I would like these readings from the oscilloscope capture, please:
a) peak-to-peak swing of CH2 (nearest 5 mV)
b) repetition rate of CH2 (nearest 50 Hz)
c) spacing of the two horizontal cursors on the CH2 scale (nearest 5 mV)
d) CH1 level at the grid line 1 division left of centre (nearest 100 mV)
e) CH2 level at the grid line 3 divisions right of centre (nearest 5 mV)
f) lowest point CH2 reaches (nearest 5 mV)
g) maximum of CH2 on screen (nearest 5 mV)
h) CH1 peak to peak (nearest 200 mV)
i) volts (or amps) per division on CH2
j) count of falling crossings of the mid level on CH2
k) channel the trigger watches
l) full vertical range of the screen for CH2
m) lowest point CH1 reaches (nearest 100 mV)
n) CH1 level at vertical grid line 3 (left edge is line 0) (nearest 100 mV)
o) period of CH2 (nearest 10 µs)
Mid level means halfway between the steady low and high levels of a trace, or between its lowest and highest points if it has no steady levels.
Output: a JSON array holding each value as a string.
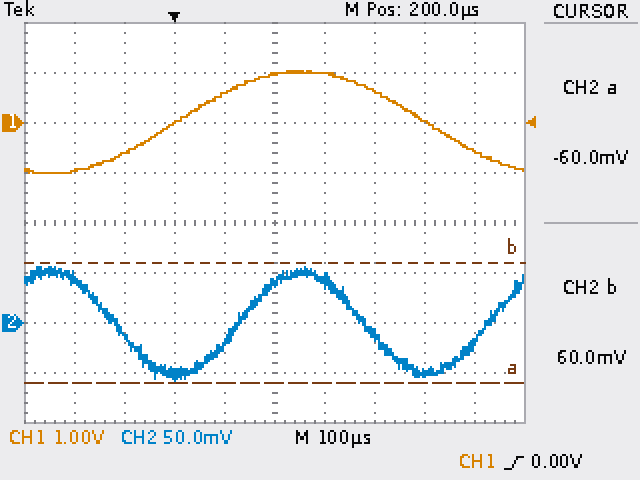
["115 mV", "2.00 kHz", "120 mV", "600 mV", "-50 mV", "-60 mV", "55 mV", "2.0 V", "50 mV", "2", "CH1", "400 mV", "-1.0 V", "0.0 V", "500 µs"]
